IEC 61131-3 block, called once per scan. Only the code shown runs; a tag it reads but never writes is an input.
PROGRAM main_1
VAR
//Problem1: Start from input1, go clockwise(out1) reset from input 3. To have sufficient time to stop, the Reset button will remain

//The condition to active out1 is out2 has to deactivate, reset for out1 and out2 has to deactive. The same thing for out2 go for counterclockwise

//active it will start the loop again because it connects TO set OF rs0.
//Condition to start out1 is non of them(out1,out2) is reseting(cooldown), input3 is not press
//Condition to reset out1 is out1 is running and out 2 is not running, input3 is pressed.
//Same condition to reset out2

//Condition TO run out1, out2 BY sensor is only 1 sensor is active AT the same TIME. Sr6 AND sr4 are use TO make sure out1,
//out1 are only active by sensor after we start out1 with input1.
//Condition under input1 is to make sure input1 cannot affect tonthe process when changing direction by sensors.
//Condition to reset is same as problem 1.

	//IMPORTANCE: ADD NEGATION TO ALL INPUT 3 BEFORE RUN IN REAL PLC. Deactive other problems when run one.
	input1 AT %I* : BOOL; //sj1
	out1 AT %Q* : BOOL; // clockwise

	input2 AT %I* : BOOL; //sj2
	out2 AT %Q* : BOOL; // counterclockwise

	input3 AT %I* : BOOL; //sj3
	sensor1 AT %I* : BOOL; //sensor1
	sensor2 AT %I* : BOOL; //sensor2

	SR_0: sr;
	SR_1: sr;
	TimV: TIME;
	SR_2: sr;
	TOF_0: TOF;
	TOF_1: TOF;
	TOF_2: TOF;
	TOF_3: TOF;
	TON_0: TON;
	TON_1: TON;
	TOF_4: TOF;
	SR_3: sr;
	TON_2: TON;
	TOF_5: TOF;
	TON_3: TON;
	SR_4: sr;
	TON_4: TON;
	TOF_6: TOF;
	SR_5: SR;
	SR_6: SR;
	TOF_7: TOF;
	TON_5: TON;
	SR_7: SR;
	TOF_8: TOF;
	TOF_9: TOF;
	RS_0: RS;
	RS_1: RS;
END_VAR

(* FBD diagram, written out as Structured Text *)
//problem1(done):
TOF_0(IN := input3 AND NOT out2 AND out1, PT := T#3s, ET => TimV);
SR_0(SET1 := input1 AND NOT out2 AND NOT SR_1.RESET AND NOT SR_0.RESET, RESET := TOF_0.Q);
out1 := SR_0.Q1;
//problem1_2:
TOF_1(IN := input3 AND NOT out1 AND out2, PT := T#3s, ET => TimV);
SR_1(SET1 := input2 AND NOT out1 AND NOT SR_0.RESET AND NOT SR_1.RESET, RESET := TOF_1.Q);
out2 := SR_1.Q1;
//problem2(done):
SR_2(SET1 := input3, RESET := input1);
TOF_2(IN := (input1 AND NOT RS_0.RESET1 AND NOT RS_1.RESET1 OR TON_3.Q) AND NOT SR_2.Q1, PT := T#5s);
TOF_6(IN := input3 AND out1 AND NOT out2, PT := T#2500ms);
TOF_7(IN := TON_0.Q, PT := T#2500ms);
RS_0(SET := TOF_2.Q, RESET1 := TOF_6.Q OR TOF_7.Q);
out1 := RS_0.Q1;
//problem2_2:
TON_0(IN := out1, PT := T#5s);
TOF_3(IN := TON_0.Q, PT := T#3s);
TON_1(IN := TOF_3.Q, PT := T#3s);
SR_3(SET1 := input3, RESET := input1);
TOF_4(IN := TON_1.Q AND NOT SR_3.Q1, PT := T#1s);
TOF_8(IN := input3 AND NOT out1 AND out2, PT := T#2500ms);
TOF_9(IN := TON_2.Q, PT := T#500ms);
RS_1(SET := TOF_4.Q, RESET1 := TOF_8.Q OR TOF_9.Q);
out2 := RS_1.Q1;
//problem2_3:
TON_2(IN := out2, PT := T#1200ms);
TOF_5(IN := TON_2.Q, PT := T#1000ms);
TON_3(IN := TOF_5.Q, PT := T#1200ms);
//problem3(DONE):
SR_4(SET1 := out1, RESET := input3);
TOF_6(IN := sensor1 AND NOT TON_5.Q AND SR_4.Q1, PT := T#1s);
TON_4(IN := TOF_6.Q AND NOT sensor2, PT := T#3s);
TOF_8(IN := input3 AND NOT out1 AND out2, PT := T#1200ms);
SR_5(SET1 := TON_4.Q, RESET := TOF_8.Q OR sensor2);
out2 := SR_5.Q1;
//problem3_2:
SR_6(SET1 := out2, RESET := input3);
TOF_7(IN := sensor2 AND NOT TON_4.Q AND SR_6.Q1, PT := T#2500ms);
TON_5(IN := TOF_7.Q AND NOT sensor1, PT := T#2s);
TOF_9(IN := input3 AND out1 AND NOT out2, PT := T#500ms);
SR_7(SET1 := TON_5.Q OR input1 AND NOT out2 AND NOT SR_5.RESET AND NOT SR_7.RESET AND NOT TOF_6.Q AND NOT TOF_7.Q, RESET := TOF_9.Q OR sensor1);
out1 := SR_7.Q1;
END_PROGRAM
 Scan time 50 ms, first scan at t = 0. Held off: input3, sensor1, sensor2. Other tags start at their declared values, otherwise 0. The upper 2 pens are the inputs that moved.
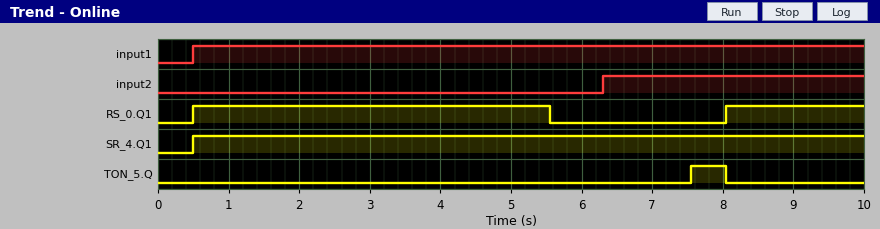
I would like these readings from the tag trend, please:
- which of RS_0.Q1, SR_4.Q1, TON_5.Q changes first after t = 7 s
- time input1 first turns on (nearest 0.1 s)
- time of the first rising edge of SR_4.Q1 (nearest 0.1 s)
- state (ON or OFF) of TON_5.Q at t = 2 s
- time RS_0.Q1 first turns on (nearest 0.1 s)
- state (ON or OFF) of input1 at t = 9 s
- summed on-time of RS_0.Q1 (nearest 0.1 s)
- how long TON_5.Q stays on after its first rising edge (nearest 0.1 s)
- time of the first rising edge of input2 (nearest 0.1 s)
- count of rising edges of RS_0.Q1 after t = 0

TON_5.Q
0.5 s
0.5 s
OFF
0.5 s
ON
7.0 s
0.5 s
6.3 s
2
